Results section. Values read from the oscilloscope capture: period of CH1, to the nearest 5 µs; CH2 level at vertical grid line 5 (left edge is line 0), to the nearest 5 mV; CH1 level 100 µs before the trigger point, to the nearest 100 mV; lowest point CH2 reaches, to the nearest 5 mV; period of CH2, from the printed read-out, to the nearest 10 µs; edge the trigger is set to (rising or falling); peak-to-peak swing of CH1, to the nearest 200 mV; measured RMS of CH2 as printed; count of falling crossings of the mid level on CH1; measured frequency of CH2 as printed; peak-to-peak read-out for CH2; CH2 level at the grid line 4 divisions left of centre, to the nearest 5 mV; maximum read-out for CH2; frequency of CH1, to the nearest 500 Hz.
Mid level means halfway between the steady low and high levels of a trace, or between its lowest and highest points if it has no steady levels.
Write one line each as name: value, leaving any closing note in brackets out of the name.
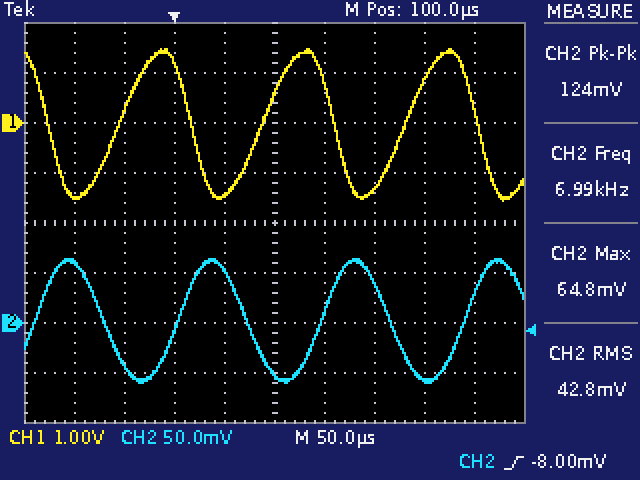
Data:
period of CH1, to the nearest 5 µs: 145 µs
CH2 level at vertical grid line 5 (left edge is line 0), to the nearest 5 mV: -50 mV
CH1 level 100 µs before the trigger point, to the nearest 100 mV: -1.5 V
lowest point CH2 reaches, to the nearest 5 mV: -60 mV
period of CH2, from the printed read-out, to the nearest 10 µs: 140 µs
edge the trigger is set to: rising
peak-to-peak swing of CH1, to the nearest 200 mV: 3.0 V
measured RMS of CH2 as printed: 42.8 mV
count of falling crossings of the mid level on CH1: 4
measured frequency of CH2 as printed: 6.99 kHz
peak-to-peak read-out for CH2: 124 mV
CH2 level at the grid line 4 divisions left of centre, to the nearest 5 mV: 60 mV
maximum read-out for CH2: 64.8 mV
frequency of CH1, to the nearest 500 Hz: 7.0 kHz
